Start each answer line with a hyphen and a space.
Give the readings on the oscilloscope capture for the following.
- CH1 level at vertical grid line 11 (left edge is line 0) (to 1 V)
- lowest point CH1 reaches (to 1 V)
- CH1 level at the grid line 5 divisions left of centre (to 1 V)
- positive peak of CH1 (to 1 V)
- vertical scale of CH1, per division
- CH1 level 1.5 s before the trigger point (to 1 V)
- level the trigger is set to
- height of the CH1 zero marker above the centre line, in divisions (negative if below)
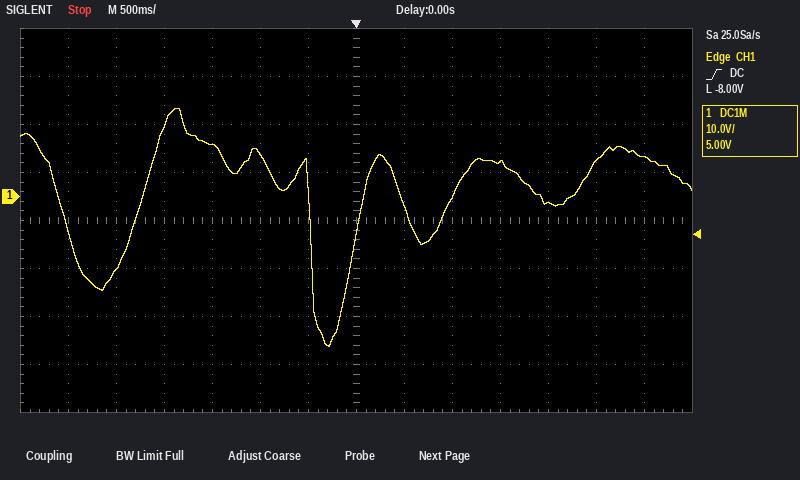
- -1 V
- -31 V
- -15 V
- 18 V
- 10 V
- 11 V
- -8.00 V
- +0.5 div
